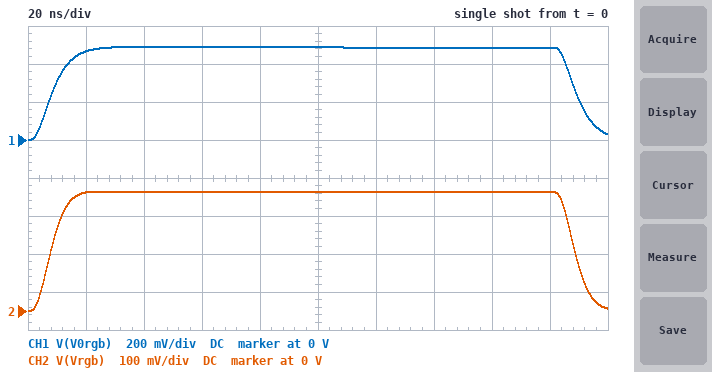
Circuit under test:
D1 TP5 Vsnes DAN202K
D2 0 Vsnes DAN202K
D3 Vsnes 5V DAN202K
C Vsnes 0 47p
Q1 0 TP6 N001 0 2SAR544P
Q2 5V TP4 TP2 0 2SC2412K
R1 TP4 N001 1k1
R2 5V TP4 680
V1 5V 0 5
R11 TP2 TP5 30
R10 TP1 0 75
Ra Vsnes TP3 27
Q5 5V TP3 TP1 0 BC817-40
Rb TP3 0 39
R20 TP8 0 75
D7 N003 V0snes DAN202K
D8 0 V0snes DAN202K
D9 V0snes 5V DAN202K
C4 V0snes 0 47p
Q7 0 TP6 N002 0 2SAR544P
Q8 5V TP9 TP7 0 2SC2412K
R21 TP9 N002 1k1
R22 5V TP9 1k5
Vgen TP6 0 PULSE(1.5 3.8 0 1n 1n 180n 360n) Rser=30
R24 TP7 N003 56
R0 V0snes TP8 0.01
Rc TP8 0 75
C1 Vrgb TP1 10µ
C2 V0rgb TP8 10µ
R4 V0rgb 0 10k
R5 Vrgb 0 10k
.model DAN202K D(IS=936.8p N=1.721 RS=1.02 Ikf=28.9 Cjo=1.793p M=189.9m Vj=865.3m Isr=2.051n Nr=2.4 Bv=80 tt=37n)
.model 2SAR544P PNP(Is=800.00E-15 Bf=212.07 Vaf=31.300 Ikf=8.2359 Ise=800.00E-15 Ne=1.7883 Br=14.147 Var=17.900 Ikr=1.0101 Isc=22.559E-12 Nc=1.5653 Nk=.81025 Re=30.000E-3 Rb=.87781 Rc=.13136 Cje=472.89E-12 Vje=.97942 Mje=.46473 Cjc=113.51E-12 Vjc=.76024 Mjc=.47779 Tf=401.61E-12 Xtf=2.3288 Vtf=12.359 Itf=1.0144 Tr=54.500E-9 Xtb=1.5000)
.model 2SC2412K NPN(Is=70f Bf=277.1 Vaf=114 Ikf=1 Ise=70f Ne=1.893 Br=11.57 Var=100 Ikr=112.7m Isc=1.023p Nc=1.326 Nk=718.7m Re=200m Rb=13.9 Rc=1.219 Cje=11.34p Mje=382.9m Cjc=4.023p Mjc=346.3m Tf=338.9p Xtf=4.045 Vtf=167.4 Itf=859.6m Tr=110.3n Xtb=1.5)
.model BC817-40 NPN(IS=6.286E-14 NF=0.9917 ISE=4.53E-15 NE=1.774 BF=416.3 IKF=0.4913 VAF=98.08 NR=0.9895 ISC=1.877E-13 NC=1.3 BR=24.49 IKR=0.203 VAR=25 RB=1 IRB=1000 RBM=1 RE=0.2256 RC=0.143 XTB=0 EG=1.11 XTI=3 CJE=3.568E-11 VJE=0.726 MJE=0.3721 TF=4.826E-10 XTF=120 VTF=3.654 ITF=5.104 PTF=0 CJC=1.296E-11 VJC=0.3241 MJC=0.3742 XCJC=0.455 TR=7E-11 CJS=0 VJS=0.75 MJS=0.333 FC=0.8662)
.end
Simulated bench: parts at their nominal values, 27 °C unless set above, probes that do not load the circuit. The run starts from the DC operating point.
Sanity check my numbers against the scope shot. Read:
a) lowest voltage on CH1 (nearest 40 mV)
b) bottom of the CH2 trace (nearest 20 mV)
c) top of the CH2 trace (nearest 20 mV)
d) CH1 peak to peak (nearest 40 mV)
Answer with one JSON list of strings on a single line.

["0 V", "0 V", "320 mV", "480 mV"]
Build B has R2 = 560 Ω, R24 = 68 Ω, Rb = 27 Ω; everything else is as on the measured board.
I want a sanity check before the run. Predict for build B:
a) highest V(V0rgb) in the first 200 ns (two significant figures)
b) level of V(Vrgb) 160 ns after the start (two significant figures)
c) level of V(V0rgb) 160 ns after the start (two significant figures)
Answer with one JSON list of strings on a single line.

["440 mV", "210 mV", "430 mV"]
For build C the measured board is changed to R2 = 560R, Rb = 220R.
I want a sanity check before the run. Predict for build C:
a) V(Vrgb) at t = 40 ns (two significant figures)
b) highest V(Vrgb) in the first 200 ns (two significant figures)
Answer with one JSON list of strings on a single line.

["570 mV", "590 mV"]
